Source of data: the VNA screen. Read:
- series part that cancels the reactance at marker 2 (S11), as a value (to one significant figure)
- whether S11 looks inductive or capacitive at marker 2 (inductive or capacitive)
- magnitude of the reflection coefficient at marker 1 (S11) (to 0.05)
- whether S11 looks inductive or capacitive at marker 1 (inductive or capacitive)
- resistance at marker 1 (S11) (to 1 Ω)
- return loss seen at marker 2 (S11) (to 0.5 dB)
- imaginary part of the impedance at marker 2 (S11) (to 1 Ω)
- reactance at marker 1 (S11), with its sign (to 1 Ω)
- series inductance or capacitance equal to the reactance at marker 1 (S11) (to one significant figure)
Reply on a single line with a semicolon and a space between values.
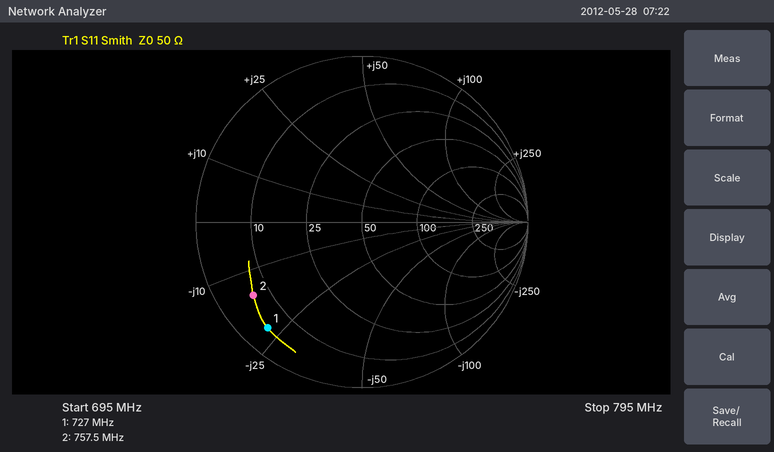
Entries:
3 nH; capacitive; 0.85; capacitive; 5 Ω; 2.0 dB; -15 Ω; -22 Ω; 10 pF
